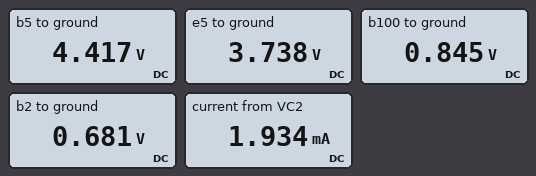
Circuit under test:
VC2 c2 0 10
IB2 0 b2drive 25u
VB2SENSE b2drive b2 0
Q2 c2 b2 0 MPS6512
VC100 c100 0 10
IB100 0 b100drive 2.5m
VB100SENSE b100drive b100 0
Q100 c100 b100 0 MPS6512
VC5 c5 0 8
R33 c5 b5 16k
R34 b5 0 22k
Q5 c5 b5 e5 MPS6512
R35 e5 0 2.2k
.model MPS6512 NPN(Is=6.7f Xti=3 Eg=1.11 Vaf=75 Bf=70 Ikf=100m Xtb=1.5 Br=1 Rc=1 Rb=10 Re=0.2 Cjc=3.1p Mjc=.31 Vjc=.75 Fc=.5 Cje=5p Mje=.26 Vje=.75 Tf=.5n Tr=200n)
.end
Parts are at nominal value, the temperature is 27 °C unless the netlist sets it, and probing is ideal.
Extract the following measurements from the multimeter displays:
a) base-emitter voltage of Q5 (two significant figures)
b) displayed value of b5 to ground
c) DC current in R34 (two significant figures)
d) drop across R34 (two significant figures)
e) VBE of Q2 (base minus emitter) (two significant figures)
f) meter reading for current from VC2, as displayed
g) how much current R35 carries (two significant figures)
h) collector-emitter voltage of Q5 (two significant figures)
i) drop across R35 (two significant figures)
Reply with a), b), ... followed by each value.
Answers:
a) 680 mV
b) 4.417 V
c) 200 µA
d) 4.4 V
e) 680 mV
f) 1.934 mA
g) 1.7 mA
h) 4.3 V
i) 3.7 V
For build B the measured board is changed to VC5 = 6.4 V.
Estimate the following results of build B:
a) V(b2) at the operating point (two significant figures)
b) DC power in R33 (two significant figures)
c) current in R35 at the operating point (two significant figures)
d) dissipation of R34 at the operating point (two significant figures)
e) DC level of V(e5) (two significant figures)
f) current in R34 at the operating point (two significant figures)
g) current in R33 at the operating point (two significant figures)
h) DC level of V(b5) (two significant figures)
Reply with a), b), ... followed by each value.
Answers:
a) 680 mV
b) 510 µW
c) 1.3 mA
d) 570 µW
e) 2.9 V
f) 160 µA
g) 180 µA
h) 3.5 V
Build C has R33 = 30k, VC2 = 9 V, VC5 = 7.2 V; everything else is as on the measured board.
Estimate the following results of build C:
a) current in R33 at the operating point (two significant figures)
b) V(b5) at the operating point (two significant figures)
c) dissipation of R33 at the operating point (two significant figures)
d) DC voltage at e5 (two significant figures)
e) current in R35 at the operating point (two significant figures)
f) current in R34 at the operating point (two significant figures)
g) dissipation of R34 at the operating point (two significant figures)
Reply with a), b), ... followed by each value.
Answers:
a) 140 µA
b) 2.9 V
c) 620 µW
d) 2.2 V
e) 1.0 mA
f) 130 µA
g) 380 µW
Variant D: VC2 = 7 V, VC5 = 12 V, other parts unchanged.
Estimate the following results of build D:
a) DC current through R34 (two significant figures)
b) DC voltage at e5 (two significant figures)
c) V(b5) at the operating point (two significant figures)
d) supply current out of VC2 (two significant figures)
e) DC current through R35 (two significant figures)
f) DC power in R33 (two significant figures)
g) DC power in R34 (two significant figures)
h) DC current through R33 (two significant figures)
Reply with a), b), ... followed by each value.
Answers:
a) 300 µA
b) 5.9 V
c) 6.6 V
d) 1.9 mA
e) 2.7 mA
f) 1.8 mW
g) 2.0 mW
h) 340 µA
